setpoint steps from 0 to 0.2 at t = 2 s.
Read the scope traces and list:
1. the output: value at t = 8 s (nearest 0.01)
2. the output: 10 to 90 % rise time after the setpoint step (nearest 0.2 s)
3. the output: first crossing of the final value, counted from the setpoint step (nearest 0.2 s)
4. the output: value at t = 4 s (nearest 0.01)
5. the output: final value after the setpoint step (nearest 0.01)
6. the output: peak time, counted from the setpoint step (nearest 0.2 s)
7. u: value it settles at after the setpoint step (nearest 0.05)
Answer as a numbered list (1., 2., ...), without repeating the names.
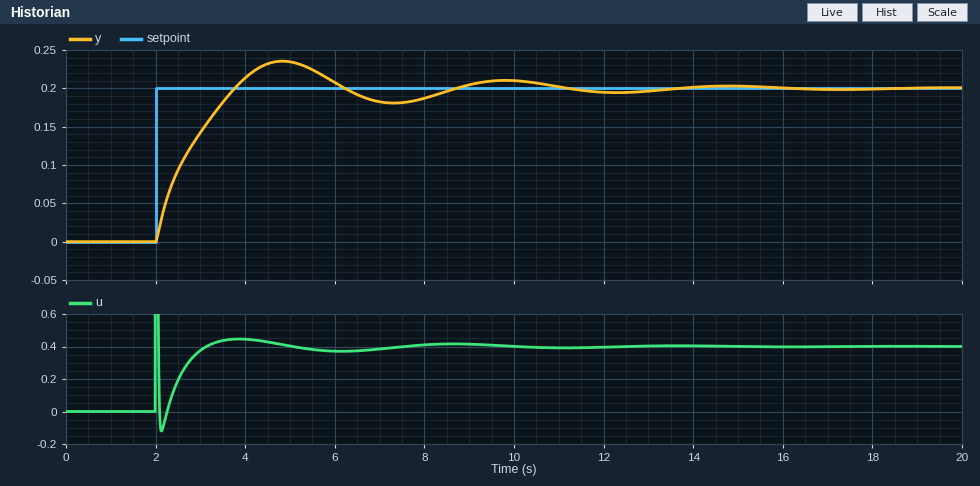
1. 0.19
2. 1.4 s
3. 1.8 s
4. 0.21
5. 0.20
6. 2.8 s
7. 0.40
